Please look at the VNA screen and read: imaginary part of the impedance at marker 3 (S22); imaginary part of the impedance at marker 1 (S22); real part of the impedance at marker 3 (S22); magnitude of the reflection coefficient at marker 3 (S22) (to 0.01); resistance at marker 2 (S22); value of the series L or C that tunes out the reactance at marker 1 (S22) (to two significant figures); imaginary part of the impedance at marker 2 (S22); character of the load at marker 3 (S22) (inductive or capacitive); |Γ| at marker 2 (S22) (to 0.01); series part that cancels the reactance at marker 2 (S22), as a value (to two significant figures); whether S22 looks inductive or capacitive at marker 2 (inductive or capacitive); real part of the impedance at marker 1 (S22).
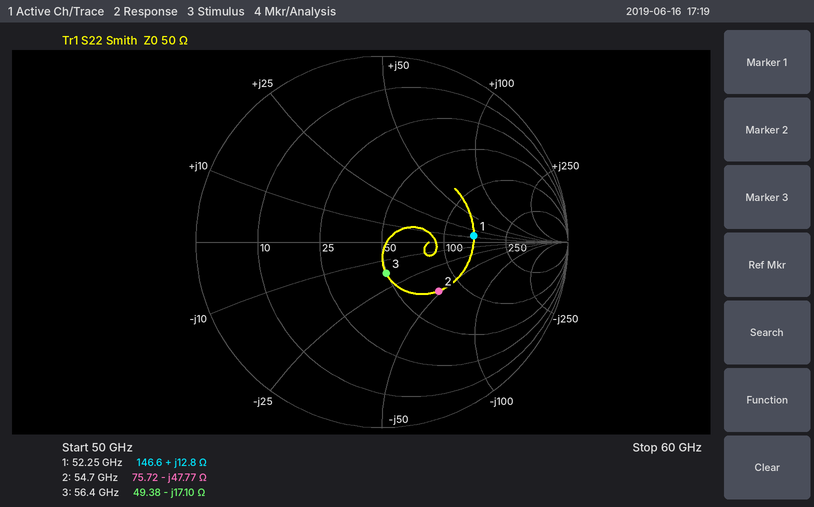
-17.10 Ω
+12.8 Ω
49.38 Ω
0.17
75.72 Ω
240 fF
-47.77 Ω
capacitive
0.40
140 pH
capacitive
146.6 Ω
